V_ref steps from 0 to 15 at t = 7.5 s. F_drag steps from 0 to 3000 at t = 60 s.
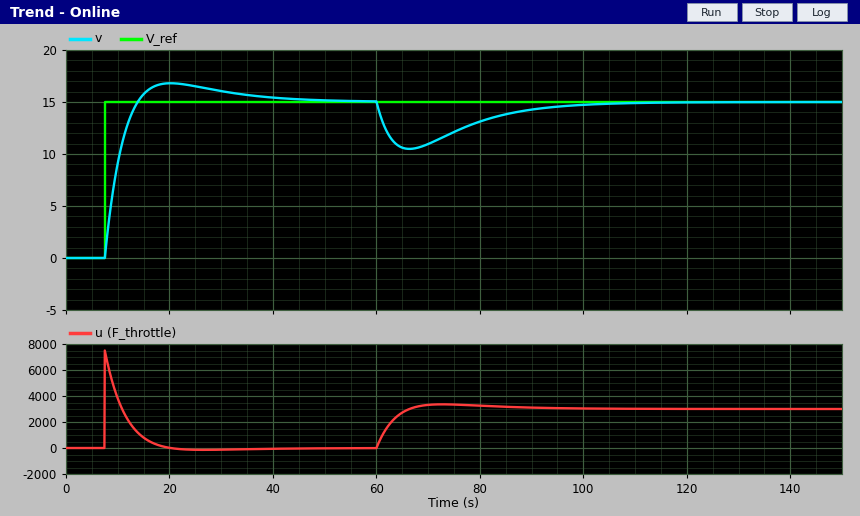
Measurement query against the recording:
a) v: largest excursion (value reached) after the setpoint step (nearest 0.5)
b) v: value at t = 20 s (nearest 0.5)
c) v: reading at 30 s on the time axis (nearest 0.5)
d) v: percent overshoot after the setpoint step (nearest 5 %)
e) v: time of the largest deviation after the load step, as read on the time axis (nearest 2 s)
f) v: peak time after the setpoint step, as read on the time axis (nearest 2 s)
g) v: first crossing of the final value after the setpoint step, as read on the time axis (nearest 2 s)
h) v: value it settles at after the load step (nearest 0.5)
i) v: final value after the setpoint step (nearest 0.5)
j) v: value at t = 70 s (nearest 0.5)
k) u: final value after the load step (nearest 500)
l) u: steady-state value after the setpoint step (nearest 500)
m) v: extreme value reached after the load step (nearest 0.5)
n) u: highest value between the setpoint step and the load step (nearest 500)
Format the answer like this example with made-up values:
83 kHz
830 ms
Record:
17.0
17.0
16.0
10 %
66 s
20 s
14 s
15.0
15.0
11.0
3000
0
10.5
7500
